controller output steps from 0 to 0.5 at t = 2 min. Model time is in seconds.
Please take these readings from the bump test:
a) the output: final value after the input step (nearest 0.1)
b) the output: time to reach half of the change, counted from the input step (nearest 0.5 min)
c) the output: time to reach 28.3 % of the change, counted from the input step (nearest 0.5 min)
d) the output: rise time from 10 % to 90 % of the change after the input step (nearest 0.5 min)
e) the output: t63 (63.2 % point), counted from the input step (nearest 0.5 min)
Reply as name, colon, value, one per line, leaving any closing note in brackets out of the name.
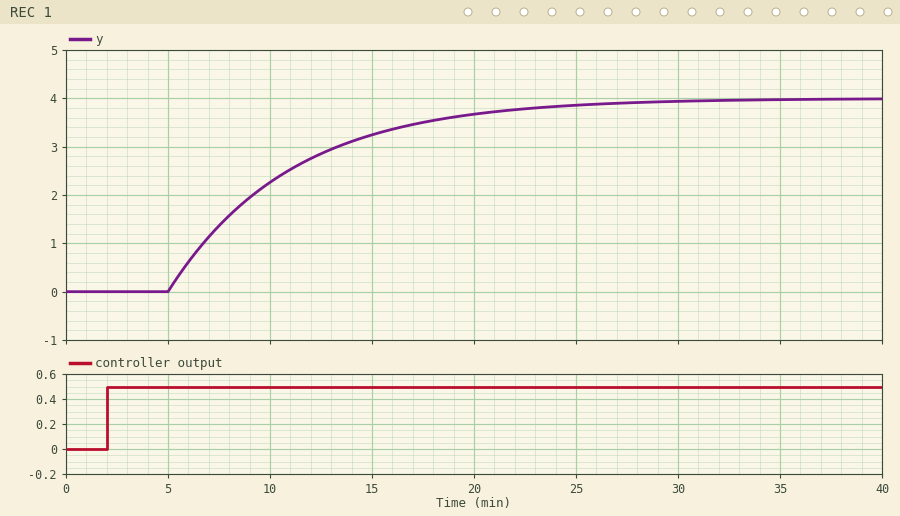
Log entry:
the output: final value after the input step: 4.0
the output: time to reach half of the change, counted from the input step: 7.0 min
the output: time to reach 28.3 % of the change, counted from the input step: 5.0 min
the output: rise time from 10 % to 90 % of the change after the input step: 13.0 min
the output: t63 (63.2 % point), counted from the input step: 9.0 min
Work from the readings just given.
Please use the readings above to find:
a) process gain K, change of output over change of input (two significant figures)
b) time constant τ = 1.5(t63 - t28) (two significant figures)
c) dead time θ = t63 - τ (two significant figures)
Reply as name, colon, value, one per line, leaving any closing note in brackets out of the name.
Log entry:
process gain K, change of output over change of input: 8.0
time constant τ = 1.5(t63 - t28): 6.0 min
dead time θ = t63 - τ: 3.0 min
